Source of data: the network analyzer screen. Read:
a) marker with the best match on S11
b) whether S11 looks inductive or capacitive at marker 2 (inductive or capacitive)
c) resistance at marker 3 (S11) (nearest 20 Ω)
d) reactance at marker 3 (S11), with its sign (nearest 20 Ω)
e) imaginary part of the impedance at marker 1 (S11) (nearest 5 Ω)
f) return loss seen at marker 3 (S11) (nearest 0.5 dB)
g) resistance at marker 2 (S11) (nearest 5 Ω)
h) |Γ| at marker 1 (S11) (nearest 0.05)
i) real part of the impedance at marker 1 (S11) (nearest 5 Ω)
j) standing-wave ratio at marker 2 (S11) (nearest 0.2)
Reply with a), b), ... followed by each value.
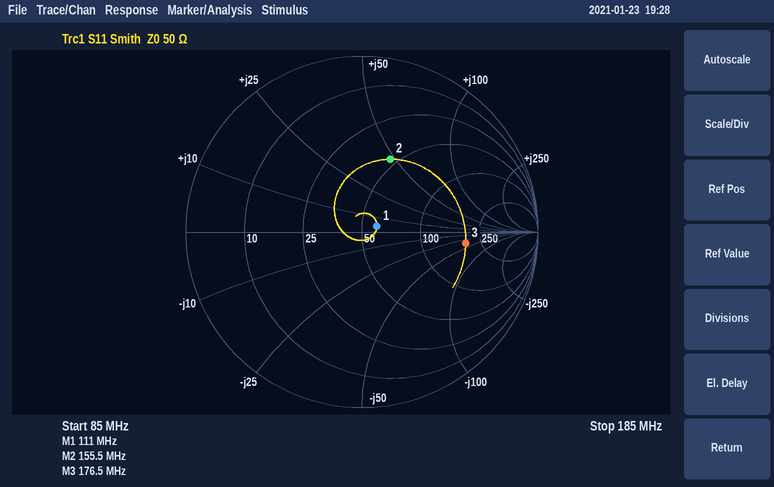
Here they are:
a) marker 1
b) inductive
c) 180 Ω
d) -40 Ω
e) +5 Ω
f) 4.5 dB
g) 45 Ω
h) 0.10
i) 60 Ω
j) 2.6
